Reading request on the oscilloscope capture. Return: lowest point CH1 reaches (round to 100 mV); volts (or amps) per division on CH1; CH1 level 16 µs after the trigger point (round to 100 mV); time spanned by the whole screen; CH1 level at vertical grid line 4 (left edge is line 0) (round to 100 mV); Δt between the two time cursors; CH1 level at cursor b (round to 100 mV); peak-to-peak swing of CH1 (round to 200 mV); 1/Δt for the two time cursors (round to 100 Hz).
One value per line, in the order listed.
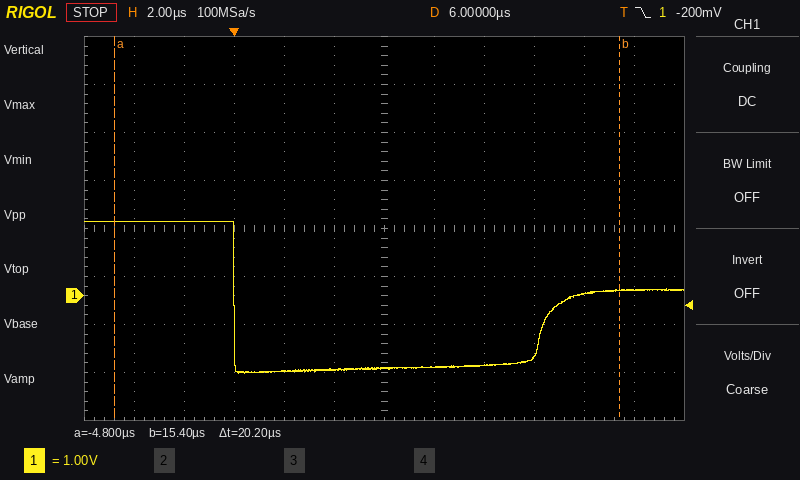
-1.6 V
1 V
100 mV
24 µs
-1.6 V
20.2 µs
100 mV
3.2 V
49.5 kHz
